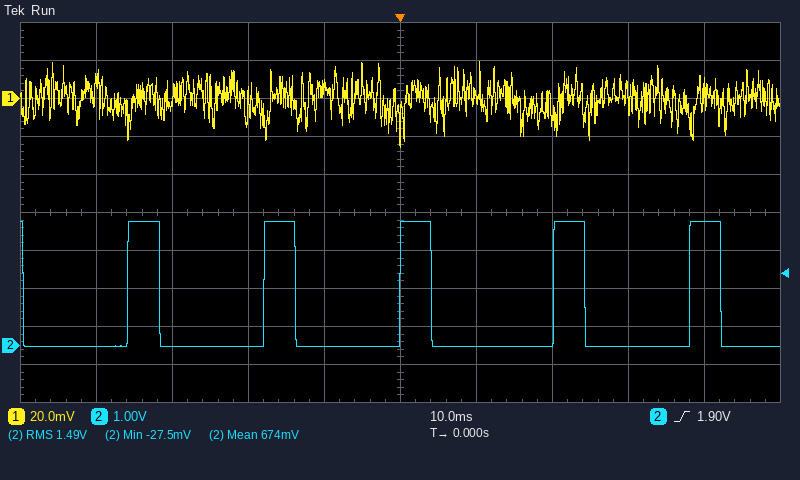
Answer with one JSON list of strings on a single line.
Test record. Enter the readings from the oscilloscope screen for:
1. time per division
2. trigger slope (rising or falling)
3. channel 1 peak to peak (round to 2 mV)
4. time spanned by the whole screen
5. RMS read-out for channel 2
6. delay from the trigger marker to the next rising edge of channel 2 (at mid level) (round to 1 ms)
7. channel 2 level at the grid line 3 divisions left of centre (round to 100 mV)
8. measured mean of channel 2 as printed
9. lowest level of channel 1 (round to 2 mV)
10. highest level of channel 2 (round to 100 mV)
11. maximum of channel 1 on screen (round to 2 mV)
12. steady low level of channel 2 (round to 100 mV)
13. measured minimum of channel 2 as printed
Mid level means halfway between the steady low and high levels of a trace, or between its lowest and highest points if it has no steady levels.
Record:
["10 ms", "rising", "46 mV", "100 ms", "1.49 V", "20 ms", "0.0 V", "674 mV", "-26 mV", "3.3 V", "20 mV", "0.0 V", "-27.5 mV"]
